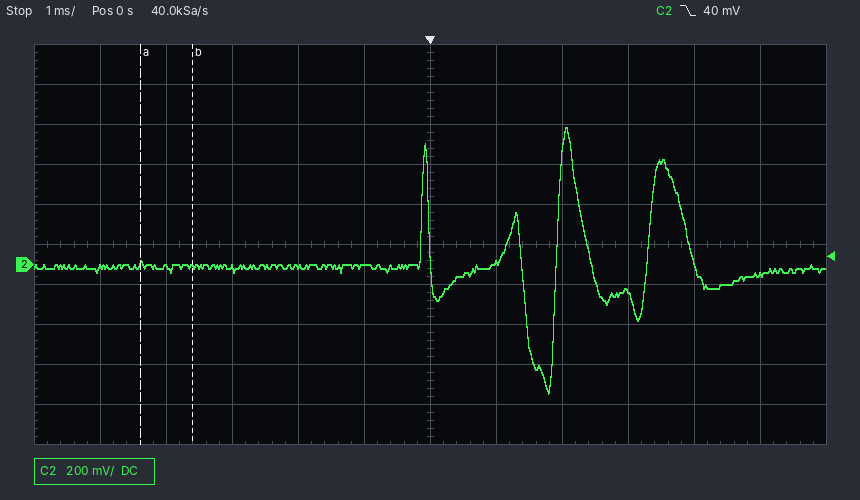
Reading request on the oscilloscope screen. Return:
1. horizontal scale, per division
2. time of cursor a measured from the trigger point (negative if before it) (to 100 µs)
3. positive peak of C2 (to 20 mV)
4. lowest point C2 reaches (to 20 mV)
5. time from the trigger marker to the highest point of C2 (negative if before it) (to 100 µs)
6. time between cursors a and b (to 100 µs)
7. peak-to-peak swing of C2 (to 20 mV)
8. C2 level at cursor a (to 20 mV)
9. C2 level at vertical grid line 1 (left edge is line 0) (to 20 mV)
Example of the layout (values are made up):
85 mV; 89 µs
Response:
1 ms; -4.4 ms; 680 mV; -640 mV; +2.1 ms; 800 µs; 1.32 V; 0 mV; -20 mV
